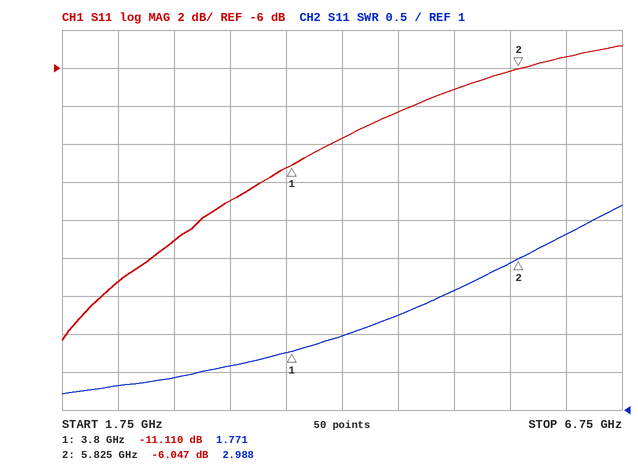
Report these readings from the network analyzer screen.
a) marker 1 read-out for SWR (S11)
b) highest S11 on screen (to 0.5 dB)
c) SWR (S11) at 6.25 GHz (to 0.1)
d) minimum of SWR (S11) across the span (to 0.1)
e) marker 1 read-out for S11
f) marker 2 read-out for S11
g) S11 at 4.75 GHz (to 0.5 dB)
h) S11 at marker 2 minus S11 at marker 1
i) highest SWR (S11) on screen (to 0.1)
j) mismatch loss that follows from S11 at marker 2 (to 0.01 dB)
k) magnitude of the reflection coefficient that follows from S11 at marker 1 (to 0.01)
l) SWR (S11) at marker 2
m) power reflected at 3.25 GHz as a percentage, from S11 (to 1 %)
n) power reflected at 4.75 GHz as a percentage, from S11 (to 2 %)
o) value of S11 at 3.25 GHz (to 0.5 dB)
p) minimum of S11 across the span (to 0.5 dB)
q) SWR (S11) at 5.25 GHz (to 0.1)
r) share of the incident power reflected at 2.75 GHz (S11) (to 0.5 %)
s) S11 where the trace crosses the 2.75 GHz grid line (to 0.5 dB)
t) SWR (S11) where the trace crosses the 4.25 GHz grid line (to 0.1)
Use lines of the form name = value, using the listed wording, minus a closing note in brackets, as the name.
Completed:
marker 1 read-out for SWR = 1.771
highest S11 on screen = -5.0 dB
SWR (S11) at 6.25 GHz = 3.3
minimum of SWR (S11) across the span = 1.2
marker 1 read-out for S11 = -11.110 dB
marker 2 read-out for S11 = -6.047 dB
S11 at 4.75 GHz = -8.5 dB
S11 at marker 2 minus S11 at marker 1 = 5.063 dB
highest SWR (S11) on screen = 3.7
mismatch loss that follows from S11 at marker 2 = 1.24 dB
magnitude of the reflection coefficient that follows from S11 at marker 1 = 0.28
SWR (S11) at marker 2 = 2.988
power reflected at 3.25 GHz as a percentage, from S11 = 5 %
power reflected at 4.75 GHz as a percentage, from S11 = 14 %
value of S11 at 3.25 GHz = -13.0 dB
minimum of S11 across the span = -20.5 dB
SWR (S11) at 5.25 GHz = 2.6
share of the incident power reflected at 2.75 GHz (S11) = 3.0 %
S11 where the trace crosses the 2.75 GHz grid line = -15.0 dB
SWR (S11) where the trace crosses the 4.25 GHz grid line = 2.0
